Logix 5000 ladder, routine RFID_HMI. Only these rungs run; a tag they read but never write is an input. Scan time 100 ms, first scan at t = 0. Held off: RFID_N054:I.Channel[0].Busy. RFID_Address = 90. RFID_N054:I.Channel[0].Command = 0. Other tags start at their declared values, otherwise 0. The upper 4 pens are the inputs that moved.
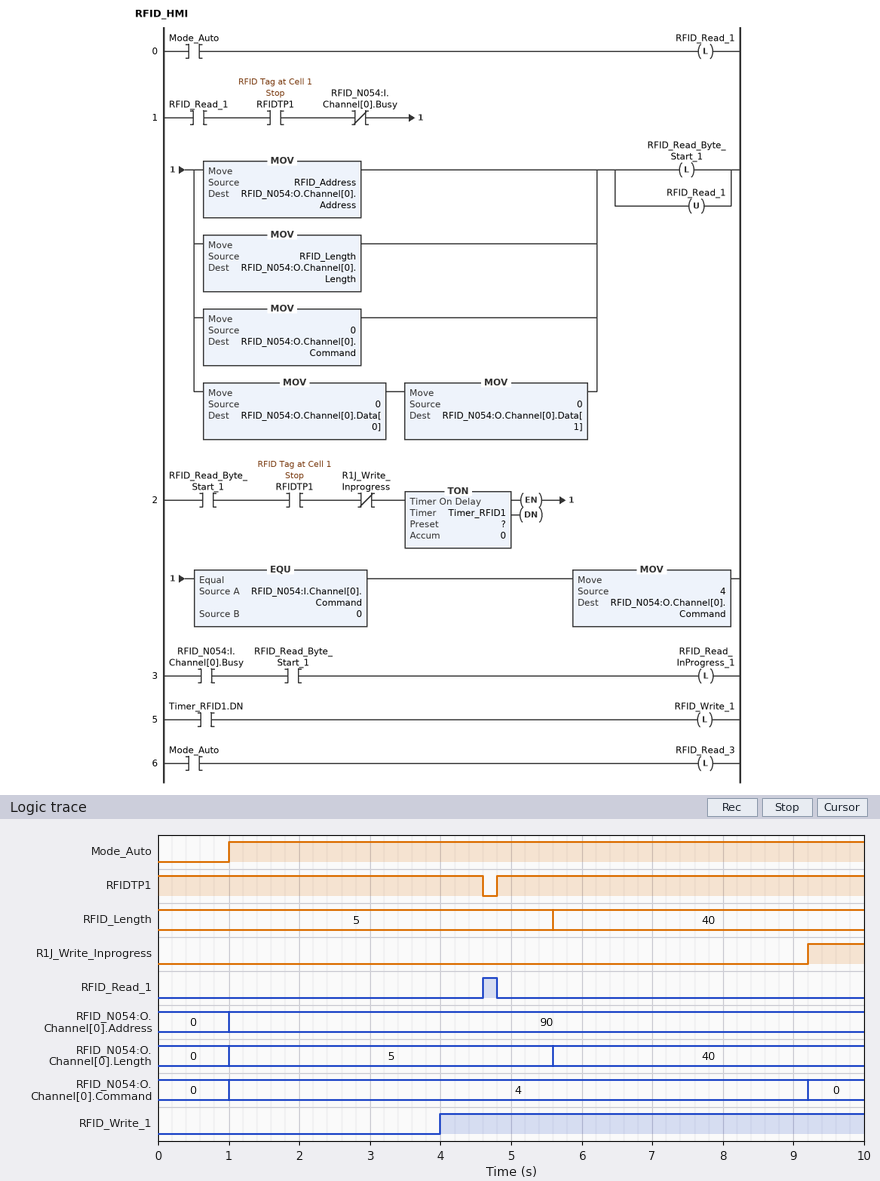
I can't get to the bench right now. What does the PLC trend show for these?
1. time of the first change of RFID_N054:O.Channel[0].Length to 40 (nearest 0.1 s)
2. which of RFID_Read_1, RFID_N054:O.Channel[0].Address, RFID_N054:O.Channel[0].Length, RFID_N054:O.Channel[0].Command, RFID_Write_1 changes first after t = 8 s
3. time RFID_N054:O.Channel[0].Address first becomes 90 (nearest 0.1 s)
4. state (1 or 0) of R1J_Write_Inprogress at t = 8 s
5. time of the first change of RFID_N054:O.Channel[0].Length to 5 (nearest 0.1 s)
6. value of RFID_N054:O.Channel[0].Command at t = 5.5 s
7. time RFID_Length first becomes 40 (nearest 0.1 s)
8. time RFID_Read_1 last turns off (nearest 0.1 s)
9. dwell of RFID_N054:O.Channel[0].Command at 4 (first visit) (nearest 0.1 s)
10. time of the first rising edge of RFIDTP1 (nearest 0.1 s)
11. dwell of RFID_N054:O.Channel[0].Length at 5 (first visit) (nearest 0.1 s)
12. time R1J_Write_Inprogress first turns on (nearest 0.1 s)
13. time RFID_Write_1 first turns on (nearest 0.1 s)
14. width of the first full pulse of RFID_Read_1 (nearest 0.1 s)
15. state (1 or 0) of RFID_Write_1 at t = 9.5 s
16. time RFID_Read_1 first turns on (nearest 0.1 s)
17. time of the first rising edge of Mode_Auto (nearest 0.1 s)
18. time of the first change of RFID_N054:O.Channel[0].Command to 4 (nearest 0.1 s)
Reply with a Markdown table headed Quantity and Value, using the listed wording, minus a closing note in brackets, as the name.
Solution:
| Quantity | Value |
|---|---|
| time of the first change of RFID_N054:O.Channel[0].Length to 40 | 5.6 s |
| which of RFID_Read_1, RFID_N054:O.Channel[0].Address, RFID_N054:O.Channel[0].Length, RFID_N054:O.Channel[0].Command, RFID_Write_1 changes first after t = 8 s | RFID_N054:O.Channel[0].Command |
| time RFID_N054:O.Channel[0].Address first becomes 90 | 1.0 s |
| state (1 or 0) of R1J_Write_Inprogress at t = 8 s | 0 |
| time of the first change of RFID_N054:O.Channel[0].Length to 5 | 1.0 s |
| value of RFID_N054:O.Channel[0].Command at t = 5.5 s | 4 |
| time RFID_Length first becomes 40 | 5.6 s |
| time RFID_Read_1 last turns off | 4.8 s |
| dwell of RFID_N054:O.Channel[0].Command at 4 (first visit) | 8.2 s |
| time of the first rising edge of RFIDTP1 | 4.8 s |
| dwell of RFID_N054:O.Channel[0].Length at 5 (first visit) | 4.6 s |
| time R1J_Write_Inprogress first turns on | 9.2 s |
| time RFID_Write_1 first turns on | 4.0 s |
| width of the first full pulse of RFID_Read_1 | 0.2 s |
| state (1 or 0) of RFID_Write_1 at t = 9.5 s | 1 |
| time RFID_Read_1 first turns on | 4.6 s |
| time of the first rising edge of Mode_Auto | 1.0 s |
| time of the first change of RFID_N054:O.Channel[0].Command to 4 | 1.0 s |
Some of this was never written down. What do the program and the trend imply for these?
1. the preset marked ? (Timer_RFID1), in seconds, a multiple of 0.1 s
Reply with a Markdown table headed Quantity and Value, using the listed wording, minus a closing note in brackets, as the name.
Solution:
| Quantity | Value |
|---|---|
| the preset marked ? (Timer_RFID1), in seconds, a multiple of 0.1 s | 3.0 s |
